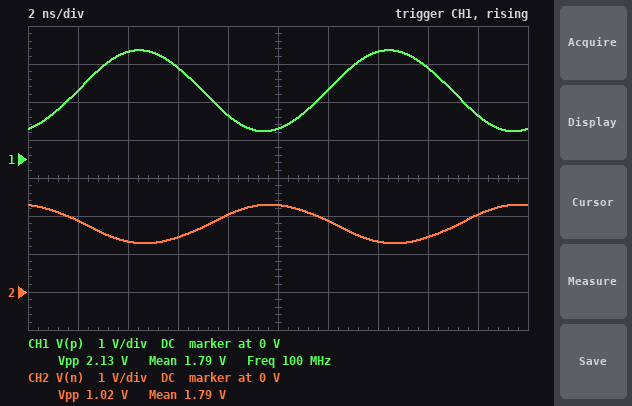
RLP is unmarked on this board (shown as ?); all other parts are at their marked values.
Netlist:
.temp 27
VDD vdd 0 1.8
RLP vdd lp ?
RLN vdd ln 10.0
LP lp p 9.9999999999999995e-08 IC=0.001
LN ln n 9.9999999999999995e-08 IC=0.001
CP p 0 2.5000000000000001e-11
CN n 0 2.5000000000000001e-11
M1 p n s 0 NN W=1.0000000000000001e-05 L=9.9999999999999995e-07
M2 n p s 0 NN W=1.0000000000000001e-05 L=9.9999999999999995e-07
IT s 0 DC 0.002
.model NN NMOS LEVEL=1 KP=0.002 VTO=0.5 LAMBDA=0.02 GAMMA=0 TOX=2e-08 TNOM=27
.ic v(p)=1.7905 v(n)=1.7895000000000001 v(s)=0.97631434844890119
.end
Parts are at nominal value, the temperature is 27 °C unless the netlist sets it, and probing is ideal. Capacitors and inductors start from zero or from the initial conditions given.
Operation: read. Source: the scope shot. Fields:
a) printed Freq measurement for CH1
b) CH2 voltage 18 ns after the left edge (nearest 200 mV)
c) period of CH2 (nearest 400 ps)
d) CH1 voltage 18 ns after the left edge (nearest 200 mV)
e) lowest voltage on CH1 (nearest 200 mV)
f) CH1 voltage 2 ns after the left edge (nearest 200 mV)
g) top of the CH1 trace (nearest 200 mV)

100 MHz
2.0 V
10.0 ns
1.2 V
800 mV
1.8 V
2.8 V
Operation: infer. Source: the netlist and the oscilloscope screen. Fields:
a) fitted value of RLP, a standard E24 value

4.7 Ω
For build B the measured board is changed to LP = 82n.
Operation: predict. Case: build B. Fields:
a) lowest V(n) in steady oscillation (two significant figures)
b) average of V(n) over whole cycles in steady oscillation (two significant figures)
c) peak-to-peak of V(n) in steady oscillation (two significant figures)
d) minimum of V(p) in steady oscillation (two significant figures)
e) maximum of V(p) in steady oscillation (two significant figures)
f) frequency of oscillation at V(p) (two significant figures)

1.4 V
1.8 V
710 mV
1.0 V
2.6 V
110 MHz
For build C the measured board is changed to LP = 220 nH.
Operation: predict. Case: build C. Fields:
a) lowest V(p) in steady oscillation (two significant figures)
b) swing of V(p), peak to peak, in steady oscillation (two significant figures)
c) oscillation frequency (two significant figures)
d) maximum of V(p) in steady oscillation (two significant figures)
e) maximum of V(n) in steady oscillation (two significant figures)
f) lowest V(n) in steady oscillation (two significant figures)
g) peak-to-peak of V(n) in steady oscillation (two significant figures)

-550 mV
4.7 V
68 MHz
4.1 V
1.9 V
1.7 V
220 mV
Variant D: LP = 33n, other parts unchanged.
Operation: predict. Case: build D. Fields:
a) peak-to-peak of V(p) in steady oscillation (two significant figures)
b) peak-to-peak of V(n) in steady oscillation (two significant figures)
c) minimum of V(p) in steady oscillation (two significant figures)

70 mV
910 mV
1.8 V
